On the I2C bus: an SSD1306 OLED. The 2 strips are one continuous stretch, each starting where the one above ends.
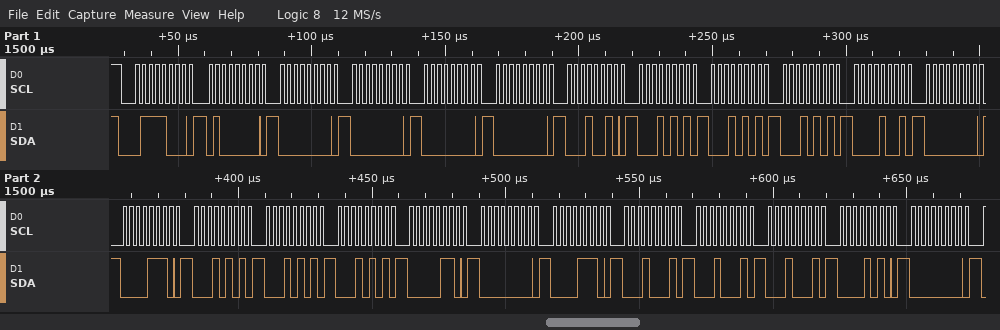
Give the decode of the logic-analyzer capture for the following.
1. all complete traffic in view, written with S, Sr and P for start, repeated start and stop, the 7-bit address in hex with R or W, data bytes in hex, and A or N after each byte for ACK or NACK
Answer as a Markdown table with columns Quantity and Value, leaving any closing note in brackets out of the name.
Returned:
| Quantity | Value |
|---|---|
| all complete traffic in view, written with S, Sr and P for start, repeated start and stop, the 7-bit address in hex with R or W, data bytes in hex, and A or N after each byte for ACK or NACK | S 3CW A 40 A 00 A 00 A 00 A 00 A 12 A 15 A 15 A 15 A 09 A 00 A 0E A 15 A 15 A 15 A 06 A 00 A 0E A 11 A 11 A 11 A 0A A 00 A |
